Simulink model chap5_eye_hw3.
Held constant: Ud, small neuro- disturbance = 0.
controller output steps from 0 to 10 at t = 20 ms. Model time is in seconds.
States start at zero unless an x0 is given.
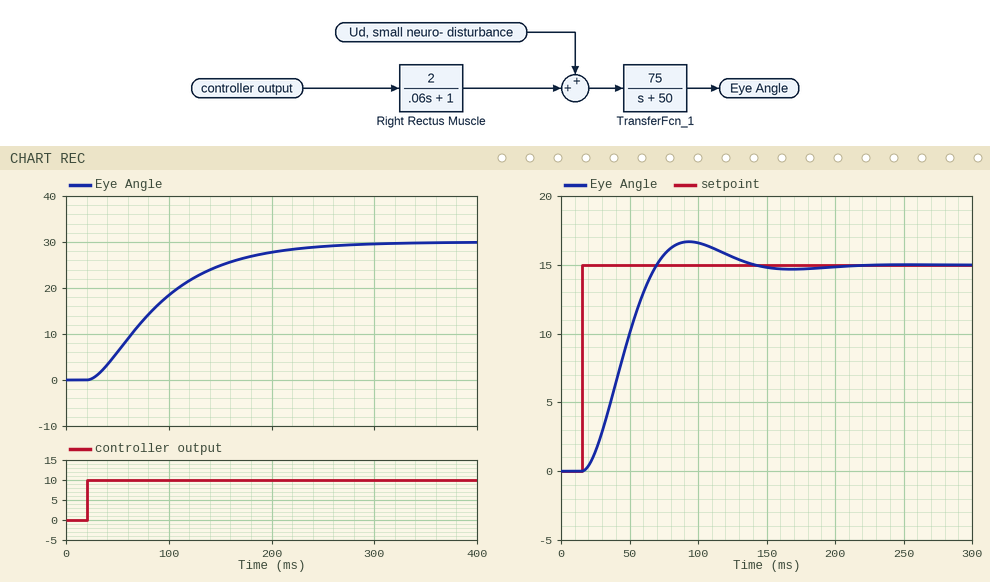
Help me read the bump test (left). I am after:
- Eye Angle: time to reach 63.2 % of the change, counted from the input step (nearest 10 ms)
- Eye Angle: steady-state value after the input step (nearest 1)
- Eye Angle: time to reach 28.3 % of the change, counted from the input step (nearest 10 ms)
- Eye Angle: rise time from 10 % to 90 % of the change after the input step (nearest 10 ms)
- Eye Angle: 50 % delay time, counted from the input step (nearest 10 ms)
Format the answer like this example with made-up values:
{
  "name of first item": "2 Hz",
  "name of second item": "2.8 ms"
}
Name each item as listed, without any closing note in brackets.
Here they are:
{
  "Eye Angle: time to reach 63.2 % of the change, counted from the input step": "80 ms",
  "Eye Angle: steady-state value after the input step": "30",
  "Eye Angle: time to reach 28.3 % of the change, counted from the input step": "40 ms",
  "Eye Angle: rise time from 10 % to 90 % of the change after the input step": "140 ms",
  "Eye Angle: 50 % delay time, counted from the input step": "60 ms"
}
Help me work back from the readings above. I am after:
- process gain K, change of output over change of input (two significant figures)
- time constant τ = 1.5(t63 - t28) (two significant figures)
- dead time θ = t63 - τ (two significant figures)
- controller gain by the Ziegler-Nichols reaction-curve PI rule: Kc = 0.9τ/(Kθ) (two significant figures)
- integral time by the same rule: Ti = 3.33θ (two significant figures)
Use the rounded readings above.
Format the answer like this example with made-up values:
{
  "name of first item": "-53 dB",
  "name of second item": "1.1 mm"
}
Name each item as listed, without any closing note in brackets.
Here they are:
{
  "process gain K, change of output over change of input": "3.0",
  "time constant τ = 1.5(t63 - t28)": "60 ms",
  "dead time θ = t63 - τ": "20 ms",
  "controller gain by the Ziegler-Nichols reaction-curve PI rule: Kc = 0.9τ/(Kθ)": "0.90",
  "integral time by the same rule: Ti = 3.33θ": "67 ms"
}
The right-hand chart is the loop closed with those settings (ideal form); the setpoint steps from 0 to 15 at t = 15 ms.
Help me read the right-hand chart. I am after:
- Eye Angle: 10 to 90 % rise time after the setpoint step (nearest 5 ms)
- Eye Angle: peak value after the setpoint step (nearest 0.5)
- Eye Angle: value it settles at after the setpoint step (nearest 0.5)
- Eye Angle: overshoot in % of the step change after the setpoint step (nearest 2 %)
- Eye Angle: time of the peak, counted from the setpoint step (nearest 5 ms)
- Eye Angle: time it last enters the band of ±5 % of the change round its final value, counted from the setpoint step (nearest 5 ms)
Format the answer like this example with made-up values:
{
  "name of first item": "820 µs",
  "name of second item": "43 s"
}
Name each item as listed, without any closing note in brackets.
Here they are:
{
  "Eye Angle: 10 to 90 % rise time after the setpoint step": "35 ms",
  "Eye Angle: peak value after the setpoint step": "16.5",
  "Eye Angle: value it settles at after the setpoint step": "15.0",
  "Eye Angle: overshoot in % of the step change after the setpoint step": "12 %",
  "Eye Angle: time of the peak, counted from the setpoint step": "80 ms",
  "Eye Angle: time it last enters the band of ±5 % of the change round its final value, counted from the setpoint step": "105 ms"
}
